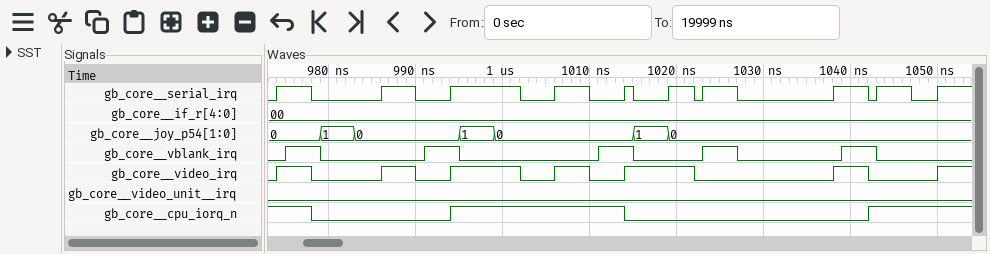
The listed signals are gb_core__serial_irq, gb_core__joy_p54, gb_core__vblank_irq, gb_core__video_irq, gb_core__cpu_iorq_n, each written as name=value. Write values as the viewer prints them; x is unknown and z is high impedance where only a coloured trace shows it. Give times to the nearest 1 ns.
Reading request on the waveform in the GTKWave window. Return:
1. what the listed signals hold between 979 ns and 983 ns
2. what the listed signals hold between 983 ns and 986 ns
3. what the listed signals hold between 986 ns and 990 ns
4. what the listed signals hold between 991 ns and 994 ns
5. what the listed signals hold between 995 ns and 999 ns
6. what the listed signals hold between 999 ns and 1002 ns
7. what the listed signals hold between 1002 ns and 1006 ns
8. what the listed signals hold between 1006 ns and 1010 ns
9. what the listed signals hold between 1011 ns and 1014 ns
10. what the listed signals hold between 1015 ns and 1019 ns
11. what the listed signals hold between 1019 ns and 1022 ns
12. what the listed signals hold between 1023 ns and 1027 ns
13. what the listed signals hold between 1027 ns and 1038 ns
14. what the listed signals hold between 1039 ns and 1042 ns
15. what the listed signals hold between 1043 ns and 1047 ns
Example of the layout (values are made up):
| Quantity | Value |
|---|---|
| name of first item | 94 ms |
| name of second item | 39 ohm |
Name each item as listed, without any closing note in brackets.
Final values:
| Quantity | Value |
|---|---|
| what the listed signals hold between 979 ns and 983 ns | gb_core__serial_irq=0, gb_core__joy_p54=1, gb_core__vblank_irq=0, gb_core__video_irq=0, gb_core__cpu_iorq_n=0 |
| what the listed signals hold between 983 ns and 986 ns | gb_core__serial_irq=0, gb_core__joy_p54=0, gb_core__vblank_irq=0, gb_core__video_irq=0, gb_core__cpu_iorq_n=0 |
| what the listed signals hold between 986 ns and 990 ns | gb_core__serial_irq=1, gb_core__joy_p54=0, gb_core__vblank_irq=0, gb_core__video_irq=1, gb_core__cpu_iorq_n=0 |
| what the listed signals hold between 991 ns and 994 ns | gb_core__serial_irq=0, gb_core__joy_p54=0, gb_core__vblank_irq=1, gb_core__video_irq=0, gb_core__cpu_iorq_n=0 |
| what the listed signals hold between 995 ns and 999 ns | gb_core__serial_irq=1, gb_core__joy_p54=1, gb_core__vblank_irq=0, gb_core__video_irq=1, gb_core__cpu_iorq_n=1 |
| what the listed signals hold between 999 ns and 1002 ns | gb_core__serial_irq=1, gb_core__joy_p54=0, gb_core__vblank_irq=0, gb_core__video_irq=1, gb_core__cpu_iorq_n=1 |
| what the listed signals hold between 1002 ns and 1006 ns | gb_core__serial_irq=0, gb_core__joy_p54=0, gb_core__vblank_irq=0, gb_core__video_irq=0, gb_core__cpu_iorq_n=1 |
| what the listed signals hold between 1006 ns and 1010 ns | gb_core__serial_irq=1, gb_core__joy_p54=0, gb_core__vblank_irq=0, gb_core__video_irq=1, gb_core__cpu_iorq_n=1 |
| what the listed signals hold between 1011 ns and 1014 ns | gb_core__serial_irq=0, gb_core__joy_p54=0, gb_core__vblank_irq=1, gb_core__video_irq=0, gb_core__cpu_iorq_n=1 |
| what the listed signals hold between 1015 ns and 1019 ns | gb_core__serial_irq=0, gb_core__joy_p54=1, gb_core__vblank_irq=0, gb_core__video_irq=1, gb_core__cpu_iorq_n=0 |
| what the listed signals hold between 1019 ns and 1022 ns | gb_core__serial_irq=1, gb_core__joy_p54=0, gb_core__vblank_irq=0, gb_core__video_irq=1, gb_core__cpu_iorq_n=0 |
| what the listed signals hold between 1023 ns and 1027 ns | gb_core__serial_irq=1, gb_core__joy_p54=0, gb_core__vblank_irq=1, gb_core__video_irq=0, gb_core__cpu_iorq_n=0 |
| what the listed signals hold between 1027 ns and 1038 ns | gb_core__serial_irq=0, gb_core__joy_p54=0, gb_core__vblank_irq=0, gb_core__video_irq=0, gb_core__cpu_iorq_n=0 |
| what the listed signals hold between 1039 ns and 1042 ns | gb_core__serial_irq=1, gb_core__joy_p54=0, gb_core__vblank_irq=1, gb_core__video_irq=1, gb_core__cpu_iorq_n=0 |
| what the listed signals hold between 1043 ns and 1047 ns | gb_core__serial_irq=1, gb_core__joy_p54=0, gb_core__vblank_irq=0, gb_core__video_irq=0, gb_core__cpu_iorq_n=1 |
